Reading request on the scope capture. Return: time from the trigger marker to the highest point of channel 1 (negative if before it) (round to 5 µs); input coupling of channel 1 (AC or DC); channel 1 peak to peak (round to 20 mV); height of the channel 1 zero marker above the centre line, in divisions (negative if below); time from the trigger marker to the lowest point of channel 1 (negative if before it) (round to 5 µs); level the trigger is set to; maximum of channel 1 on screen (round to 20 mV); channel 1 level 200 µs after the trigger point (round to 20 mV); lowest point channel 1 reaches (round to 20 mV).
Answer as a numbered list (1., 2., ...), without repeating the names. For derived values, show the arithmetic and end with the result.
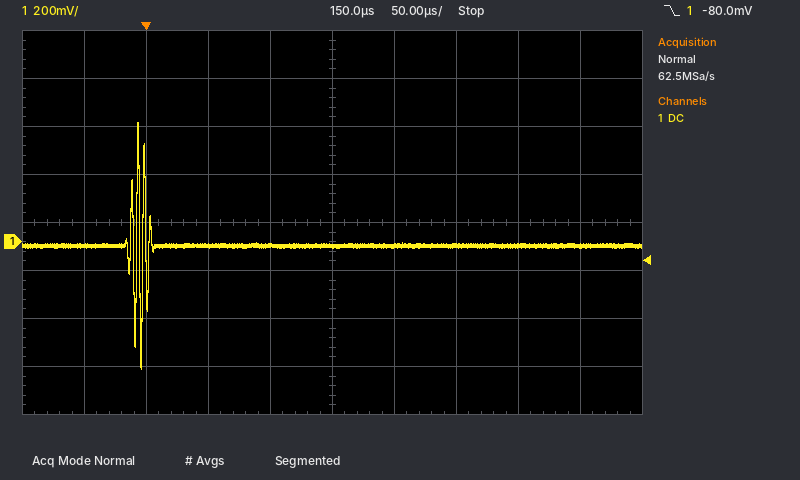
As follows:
1. -5 µs
2. DC
3. 500 mV − (-520 mV) = 1.02 V
4. -0.4 div
5. -5 µs
6. -80.0 mV
7. 500 mV
8. -20 mV
9. -520 mV
